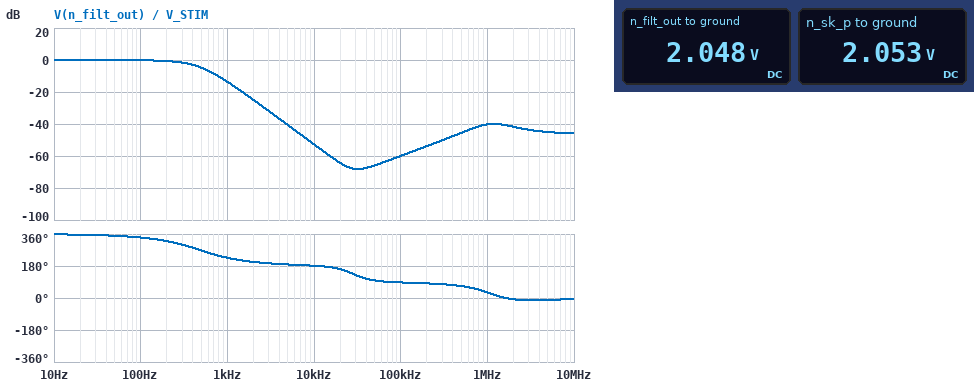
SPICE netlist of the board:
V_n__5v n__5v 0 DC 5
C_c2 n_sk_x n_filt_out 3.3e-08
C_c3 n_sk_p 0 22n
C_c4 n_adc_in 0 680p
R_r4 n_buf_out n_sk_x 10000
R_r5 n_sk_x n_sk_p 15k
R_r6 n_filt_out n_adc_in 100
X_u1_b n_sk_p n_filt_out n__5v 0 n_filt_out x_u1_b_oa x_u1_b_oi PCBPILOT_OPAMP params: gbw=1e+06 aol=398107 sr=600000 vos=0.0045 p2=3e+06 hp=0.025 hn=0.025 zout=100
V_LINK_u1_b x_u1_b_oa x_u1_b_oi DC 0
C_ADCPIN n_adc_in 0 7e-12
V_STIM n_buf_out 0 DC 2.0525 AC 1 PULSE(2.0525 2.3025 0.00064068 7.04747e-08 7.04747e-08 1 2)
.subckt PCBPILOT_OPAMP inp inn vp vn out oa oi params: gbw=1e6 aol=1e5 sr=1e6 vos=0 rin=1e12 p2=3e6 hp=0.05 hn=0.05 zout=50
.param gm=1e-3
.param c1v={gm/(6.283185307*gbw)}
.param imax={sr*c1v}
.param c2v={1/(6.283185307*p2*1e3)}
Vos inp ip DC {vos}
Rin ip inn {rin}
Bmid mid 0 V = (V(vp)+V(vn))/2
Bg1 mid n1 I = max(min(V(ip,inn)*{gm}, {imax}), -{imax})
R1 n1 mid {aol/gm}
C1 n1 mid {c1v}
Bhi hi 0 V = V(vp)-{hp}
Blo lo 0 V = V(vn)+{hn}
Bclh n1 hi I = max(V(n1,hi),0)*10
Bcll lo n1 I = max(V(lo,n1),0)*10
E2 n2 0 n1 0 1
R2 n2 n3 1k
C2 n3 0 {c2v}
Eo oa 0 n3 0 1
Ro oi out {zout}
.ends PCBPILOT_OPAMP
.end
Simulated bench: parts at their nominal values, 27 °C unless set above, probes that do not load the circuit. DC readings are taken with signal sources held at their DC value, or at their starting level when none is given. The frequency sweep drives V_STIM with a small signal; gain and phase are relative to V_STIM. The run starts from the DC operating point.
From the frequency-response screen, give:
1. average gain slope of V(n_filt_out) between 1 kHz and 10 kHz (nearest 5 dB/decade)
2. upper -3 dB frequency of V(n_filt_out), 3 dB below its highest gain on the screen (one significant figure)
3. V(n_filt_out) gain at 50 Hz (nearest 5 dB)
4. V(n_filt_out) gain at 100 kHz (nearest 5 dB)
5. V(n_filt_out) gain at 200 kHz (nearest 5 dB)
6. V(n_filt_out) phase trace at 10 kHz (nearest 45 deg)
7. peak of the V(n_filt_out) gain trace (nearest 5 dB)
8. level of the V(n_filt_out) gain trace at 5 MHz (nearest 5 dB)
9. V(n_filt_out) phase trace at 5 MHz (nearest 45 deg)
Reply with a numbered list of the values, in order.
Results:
1. -40 dB/decade
2. 400 Hz
3. 0 dB
4. -60 dB
5. -55 dB
6. 180 deg
7. 0 dB
8. -45 dB
9. 0 deg
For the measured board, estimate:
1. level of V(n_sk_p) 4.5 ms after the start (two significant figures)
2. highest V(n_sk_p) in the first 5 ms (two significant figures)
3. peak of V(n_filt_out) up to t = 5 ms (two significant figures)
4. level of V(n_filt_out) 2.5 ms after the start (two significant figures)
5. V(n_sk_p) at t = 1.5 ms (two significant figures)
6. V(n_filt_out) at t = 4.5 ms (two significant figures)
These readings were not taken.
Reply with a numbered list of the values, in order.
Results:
1. 2.3 V
2. 2.3 V
3. 2.3 V
4. 2.3 V
5. 2.3 V
6. 2.3 V
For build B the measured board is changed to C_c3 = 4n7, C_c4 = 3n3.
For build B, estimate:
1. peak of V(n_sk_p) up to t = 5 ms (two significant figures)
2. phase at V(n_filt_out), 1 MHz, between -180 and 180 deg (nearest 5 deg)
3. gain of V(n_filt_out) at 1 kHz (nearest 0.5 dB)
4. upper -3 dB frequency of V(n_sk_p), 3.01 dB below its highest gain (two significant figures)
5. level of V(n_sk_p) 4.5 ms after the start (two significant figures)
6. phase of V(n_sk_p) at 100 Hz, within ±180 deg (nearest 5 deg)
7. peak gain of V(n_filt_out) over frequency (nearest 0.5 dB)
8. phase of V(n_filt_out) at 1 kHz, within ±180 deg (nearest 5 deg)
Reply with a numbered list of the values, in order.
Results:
1. 2.4 V
2. 20 deg
3. 2.5 dB
4. 1.2 kHz
5. 2.3 V
6. -5 deg
7. 3.0 dB
8. -85 deg
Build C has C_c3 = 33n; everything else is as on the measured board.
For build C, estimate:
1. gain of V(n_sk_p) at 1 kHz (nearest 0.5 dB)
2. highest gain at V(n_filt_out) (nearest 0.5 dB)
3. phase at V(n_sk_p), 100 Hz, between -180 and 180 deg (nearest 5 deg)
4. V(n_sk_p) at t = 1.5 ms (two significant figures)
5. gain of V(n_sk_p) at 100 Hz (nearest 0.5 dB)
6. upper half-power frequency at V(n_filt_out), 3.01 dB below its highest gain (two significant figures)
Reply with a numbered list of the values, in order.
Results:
1. -17.5 dB
2. 0 dB
3. -30 deg
4. 2.2 V
5. -0.5 dB
6. 250 Hz
